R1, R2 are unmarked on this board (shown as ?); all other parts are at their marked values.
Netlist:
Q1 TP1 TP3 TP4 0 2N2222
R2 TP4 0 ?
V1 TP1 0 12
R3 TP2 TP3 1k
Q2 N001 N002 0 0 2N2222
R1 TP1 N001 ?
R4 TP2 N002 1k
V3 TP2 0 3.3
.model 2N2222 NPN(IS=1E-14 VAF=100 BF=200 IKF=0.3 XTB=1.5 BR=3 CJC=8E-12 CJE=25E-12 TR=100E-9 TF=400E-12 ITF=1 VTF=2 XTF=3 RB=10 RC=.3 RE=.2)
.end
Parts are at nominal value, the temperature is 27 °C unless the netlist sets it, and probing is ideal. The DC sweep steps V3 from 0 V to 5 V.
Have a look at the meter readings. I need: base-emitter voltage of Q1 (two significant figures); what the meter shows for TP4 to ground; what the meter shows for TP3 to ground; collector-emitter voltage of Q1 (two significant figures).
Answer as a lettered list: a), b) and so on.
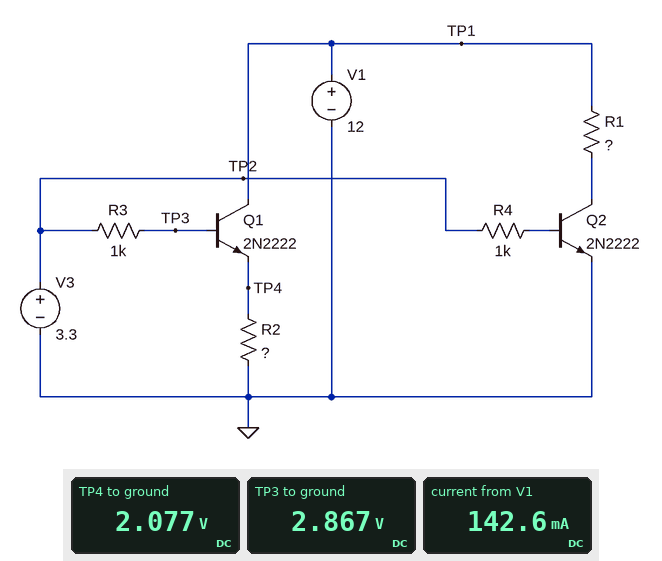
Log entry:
a) 790 mV
b) 2.077 V
c) 2.867 V
d) 9.9 V
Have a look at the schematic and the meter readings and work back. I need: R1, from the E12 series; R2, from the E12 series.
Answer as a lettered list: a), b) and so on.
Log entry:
a) 180 Ω
b) 27 Ω
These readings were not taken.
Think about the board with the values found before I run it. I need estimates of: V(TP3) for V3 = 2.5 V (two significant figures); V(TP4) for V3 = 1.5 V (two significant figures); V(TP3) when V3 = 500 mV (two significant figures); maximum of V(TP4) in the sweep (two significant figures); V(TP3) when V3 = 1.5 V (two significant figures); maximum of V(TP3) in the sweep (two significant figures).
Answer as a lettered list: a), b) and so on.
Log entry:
a) 2.2 V
b) 640 mV
c) 500 mV
d) 3.4 V
e) 1.4 V
f) 4.2 V
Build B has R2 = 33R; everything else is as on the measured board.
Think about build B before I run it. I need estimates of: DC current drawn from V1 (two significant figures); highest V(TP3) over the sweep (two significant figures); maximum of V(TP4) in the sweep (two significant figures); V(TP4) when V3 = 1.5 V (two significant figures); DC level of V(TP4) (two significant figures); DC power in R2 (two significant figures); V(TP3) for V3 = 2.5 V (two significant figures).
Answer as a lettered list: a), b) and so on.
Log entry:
a) 130 mA
b) 4.3 V
c) 3.5 V
d) 670 mV
e) 2.2 V
f) 140 mW
g) 2.3 V
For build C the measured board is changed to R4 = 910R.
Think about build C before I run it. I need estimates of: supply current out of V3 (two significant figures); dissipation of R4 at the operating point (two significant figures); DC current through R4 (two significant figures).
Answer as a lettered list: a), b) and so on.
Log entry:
a) 3.2 mA
b) 6.8 mW
c) 2.7 mA
